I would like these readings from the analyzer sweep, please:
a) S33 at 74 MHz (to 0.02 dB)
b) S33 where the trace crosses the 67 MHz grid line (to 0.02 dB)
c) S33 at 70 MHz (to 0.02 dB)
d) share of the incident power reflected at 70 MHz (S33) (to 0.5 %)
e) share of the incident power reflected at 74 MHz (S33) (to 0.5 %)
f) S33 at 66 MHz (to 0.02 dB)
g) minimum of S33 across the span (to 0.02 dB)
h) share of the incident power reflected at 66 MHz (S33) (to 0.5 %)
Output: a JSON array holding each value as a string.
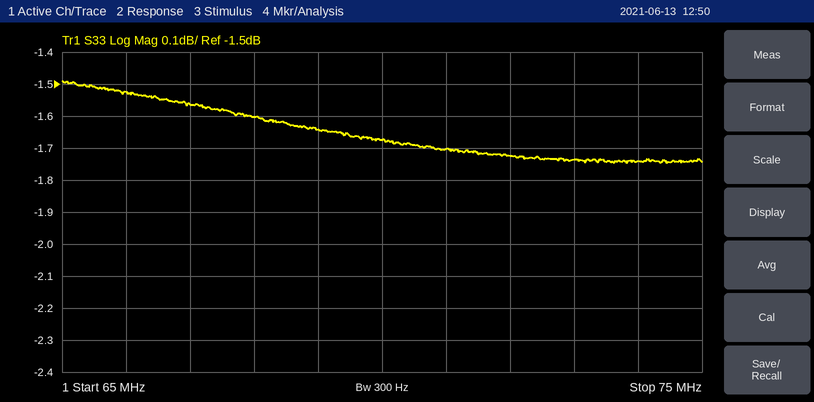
["-1.74 dB", "-1.56 dB", "-1.68 dB", "68.0 %", "67.0 %", "-1.52 dB", "-1.74 dB", "70.5 %"]
